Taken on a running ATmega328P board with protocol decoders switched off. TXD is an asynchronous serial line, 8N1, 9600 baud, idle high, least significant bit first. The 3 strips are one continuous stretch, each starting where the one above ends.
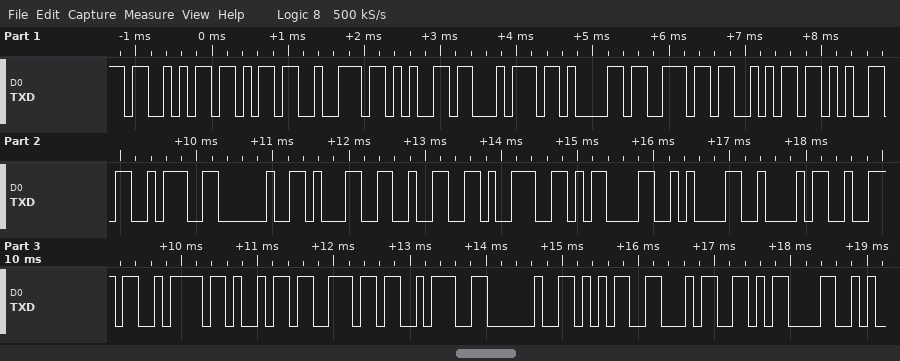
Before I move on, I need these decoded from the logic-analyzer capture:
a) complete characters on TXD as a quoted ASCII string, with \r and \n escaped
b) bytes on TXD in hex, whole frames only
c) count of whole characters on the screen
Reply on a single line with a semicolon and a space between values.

"Skretanje: 129\r\nBrzin: 54\r"; 53 6B 72 65 74 61 6E 6A 65 3A 20 31 32 39 0D 0A 42 72 7A 69 6E 3A 20 35 34 0D; 26
